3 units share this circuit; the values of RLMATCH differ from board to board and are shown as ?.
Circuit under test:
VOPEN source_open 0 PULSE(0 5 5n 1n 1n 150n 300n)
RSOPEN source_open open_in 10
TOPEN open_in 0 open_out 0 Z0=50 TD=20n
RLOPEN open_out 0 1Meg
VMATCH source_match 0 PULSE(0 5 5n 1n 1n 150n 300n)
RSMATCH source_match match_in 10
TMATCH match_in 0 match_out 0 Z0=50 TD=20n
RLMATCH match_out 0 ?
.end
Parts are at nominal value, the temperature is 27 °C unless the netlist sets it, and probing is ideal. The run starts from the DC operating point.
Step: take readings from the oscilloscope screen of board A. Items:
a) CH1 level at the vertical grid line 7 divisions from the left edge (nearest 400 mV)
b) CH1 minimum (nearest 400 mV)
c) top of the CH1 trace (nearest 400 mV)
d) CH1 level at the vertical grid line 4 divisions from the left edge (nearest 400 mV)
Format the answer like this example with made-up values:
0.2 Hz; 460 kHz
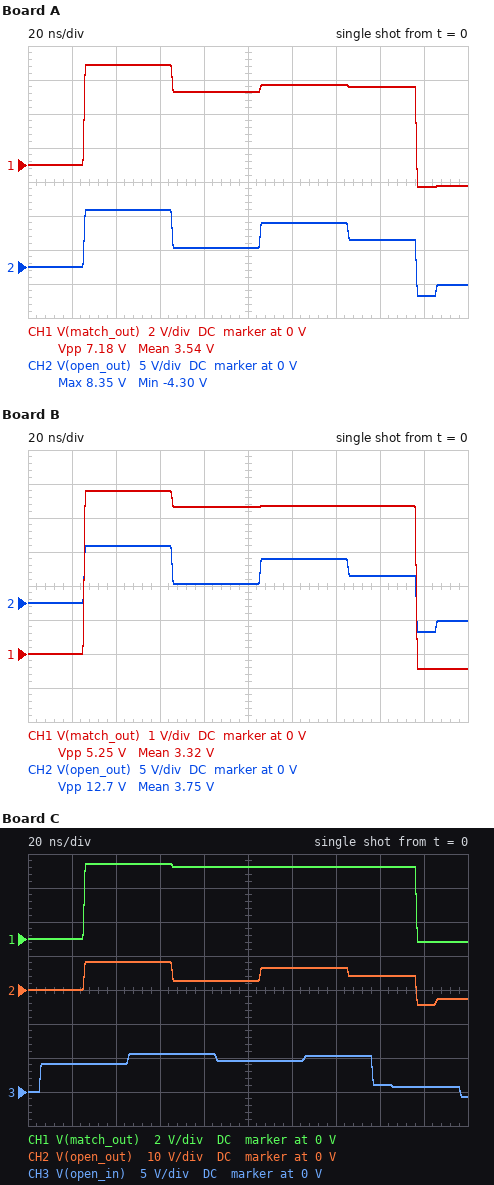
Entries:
4.8 V; -1.2 V; 6.0 V; 4.4 V
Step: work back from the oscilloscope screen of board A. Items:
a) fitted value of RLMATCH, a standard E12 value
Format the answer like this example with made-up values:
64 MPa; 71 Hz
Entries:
120 Ω
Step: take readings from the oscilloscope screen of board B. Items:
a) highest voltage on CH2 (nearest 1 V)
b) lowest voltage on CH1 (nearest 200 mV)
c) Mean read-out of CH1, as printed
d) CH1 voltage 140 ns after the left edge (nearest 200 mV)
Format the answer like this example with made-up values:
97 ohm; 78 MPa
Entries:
8 V; -400 mV; 3.32 V; 4.4 V
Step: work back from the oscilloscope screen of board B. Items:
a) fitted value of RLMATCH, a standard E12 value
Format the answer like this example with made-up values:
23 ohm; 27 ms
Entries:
68 Ω
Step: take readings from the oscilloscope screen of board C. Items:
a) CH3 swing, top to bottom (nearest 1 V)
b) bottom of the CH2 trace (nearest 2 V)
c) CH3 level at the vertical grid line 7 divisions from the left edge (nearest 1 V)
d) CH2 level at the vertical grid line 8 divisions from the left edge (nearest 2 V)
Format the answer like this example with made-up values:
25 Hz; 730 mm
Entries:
6 V; -4 V; 5 V; 4 V
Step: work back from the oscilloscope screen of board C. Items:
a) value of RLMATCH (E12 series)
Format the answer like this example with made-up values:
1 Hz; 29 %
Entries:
56 Ω
